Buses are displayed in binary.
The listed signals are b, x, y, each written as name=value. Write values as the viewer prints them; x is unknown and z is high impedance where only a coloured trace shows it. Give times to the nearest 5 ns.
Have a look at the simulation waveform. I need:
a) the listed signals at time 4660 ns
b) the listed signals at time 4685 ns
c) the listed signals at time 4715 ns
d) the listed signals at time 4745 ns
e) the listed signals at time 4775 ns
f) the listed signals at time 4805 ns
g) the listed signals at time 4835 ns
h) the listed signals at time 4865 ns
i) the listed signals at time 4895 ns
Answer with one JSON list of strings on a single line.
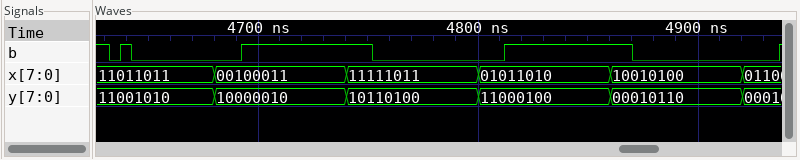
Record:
["b=0, x=11011011, y=11001010", "b=0, x=00100011, y=10000010", "b=1, x=00100011, y=10000010", "b=1, x=11111011, y=10110100", "b=0, x=11111011, y=10110100", "b=0, x=01011010, y=11000100", "b=1, x=01011010, y=11000100", "b=1, x=10010100, y=00010110", "b=0, x=10010100, y=00010110"]
